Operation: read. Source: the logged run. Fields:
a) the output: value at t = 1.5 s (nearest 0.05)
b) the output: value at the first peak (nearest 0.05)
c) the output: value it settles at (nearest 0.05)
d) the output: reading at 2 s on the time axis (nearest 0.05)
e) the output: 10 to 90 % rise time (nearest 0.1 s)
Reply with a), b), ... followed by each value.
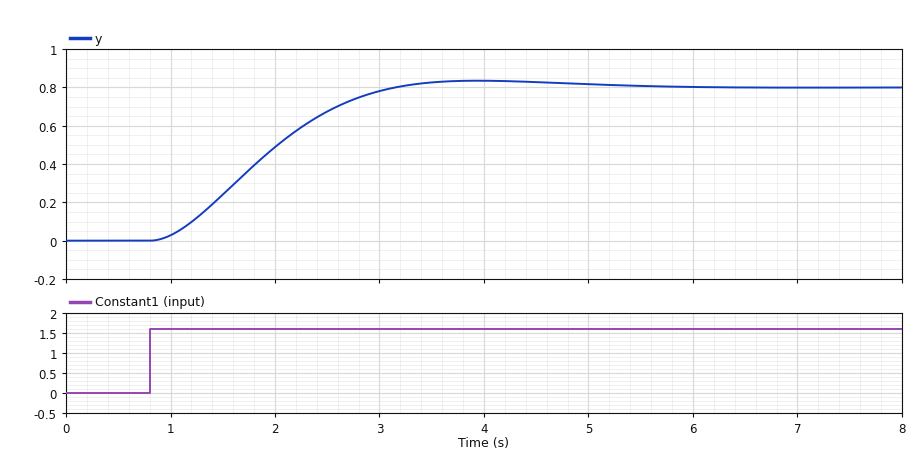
a) 0.25
b) 0.85
c) 0.80
d) 0.50
e) 1.5 s
